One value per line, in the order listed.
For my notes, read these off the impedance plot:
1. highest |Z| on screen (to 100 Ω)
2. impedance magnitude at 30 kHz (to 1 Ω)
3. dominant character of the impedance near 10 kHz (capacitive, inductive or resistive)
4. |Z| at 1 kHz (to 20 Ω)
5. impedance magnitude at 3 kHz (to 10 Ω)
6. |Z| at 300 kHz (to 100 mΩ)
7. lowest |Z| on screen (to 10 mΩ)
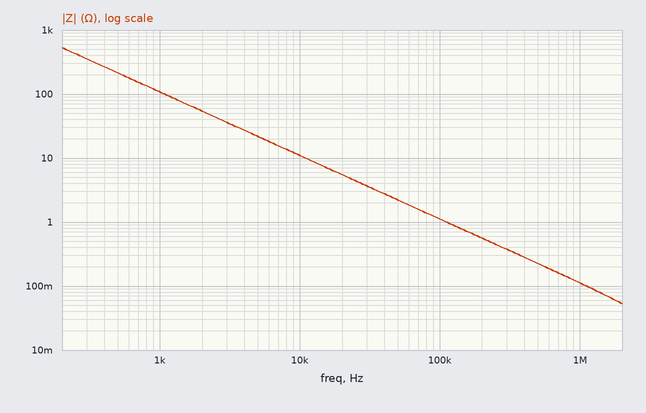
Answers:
500 Ω
4 Ω
capacitive
100 Ω
40 Ω
400 mΩ
50 mΩ
